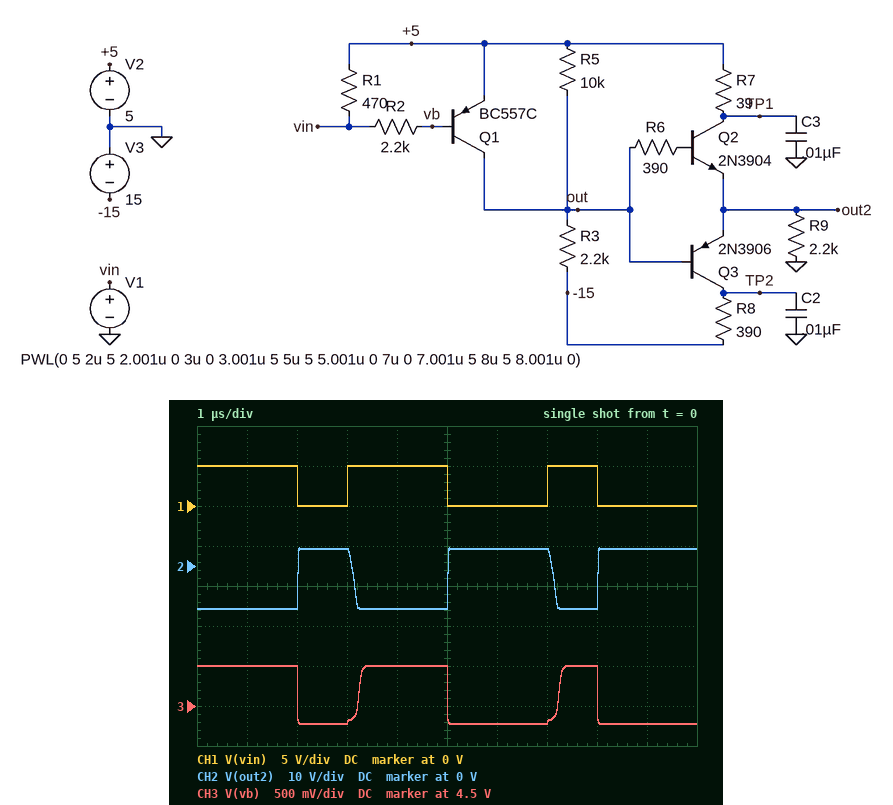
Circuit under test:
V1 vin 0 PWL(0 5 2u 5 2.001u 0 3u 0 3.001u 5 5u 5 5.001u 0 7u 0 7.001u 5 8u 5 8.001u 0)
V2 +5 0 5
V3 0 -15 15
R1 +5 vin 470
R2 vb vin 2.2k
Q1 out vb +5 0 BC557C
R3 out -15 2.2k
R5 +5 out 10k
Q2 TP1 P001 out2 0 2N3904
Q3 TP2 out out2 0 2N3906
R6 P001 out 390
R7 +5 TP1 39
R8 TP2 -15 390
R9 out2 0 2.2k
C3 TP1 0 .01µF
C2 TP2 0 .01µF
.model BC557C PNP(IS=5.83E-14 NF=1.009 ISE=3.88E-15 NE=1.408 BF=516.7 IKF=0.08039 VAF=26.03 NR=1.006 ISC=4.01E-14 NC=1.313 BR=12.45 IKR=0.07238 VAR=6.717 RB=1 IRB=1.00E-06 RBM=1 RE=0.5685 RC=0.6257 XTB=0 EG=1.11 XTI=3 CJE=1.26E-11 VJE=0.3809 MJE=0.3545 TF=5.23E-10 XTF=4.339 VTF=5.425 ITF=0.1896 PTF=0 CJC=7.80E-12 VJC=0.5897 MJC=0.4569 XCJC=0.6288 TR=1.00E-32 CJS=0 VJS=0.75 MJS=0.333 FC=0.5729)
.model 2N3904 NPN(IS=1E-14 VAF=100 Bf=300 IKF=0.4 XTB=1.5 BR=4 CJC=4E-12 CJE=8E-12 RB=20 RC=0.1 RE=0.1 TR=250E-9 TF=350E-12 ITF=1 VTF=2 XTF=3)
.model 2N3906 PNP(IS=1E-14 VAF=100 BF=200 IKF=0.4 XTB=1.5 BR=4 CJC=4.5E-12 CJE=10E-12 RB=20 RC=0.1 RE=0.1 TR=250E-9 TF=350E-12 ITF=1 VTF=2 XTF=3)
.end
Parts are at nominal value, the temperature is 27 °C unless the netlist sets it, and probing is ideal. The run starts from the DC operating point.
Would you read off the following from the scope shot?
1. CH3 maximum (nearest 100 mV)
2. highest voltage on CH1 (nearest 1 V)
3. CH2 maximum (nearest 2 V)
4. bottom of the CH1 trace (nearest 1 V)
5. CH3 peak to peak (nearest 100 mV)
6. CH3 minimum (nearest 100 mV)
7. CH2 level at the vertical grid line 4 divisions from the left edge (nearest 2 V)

5.0 V
5 V
4 V
0 V
700 mV
4.3 V
-10 V
